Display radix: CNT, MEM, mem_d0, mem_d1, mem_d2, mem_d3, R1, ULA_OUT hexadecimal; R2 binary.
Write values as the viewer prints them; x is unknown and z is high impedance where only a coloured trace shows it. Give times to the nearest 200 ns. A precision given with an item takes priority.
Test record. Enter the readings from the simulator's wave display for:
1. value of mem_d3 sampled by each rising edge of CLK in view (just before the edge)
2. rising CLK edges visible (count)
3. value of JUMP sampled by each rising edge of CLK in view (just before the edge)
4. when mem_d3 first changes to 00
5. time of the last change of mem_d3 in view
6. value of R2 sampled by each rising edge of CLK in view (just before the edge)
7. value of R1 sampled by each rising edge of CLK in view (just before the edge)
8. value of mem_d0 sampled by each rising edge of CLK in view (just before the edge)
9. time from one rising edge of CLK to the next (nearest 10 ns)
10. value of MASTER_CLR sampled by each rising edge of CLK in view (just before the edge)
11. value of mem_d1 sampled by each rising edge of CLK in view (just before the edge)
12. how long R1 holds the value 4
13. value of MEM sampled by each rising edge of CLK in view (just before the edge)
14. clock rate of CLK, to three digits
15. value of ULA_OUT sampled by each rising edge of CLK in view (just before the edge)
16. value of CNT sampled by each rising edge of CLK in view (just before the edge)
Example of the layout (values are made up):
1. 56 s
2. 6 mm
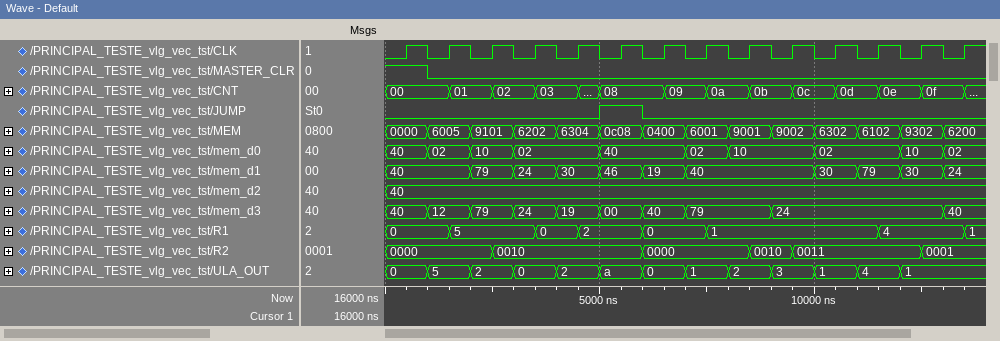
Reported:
1. 40, 12, 79, 24, 19, 00, 40, 79, 79, 24, 24, 24, 24, 40
2. 14
3. 0 0 0 0 0 1 0 0 0 0 0 0 0 0
4. 5000 ns
5. 13000 ns
6. 0000, 0000, 0000, 0010, 0010, 0010, 0000, 0000, 0000, 0010, 0011, 0011, 0011, 0001
7. 0, 0, 5, 5, 0, 2, 0, 0, 1, 1, 1, 1, 4, 4
8. 40, 02, 10, 02, 02, 40, 40, 02, 10, 10, 02, 02, 10, 02
9. 1000 ns
10. 1 0 0 0 0 0 0 0 0 0 0 0 0 0
11. 40, 40, 79, 24, 30, 46, 19, 40, 40, 40, 30, 79, 30, 24
12. 2000 ns
13. 0000, 6005, 9101, 6202, 6304, 0c08, 0400, 6001, 9001, 9002, 6302, 6102, 9302, 6200
14. 1.00 MHz
15. 0, 5, 2, 0, 2, a, 0, 1, 2, 3, 1, 4, 1, 1
16. 00, 00, 01, 02, 03, 08, 08, 09, 0a, 0b, 0c, 0d, 0e, 0f
